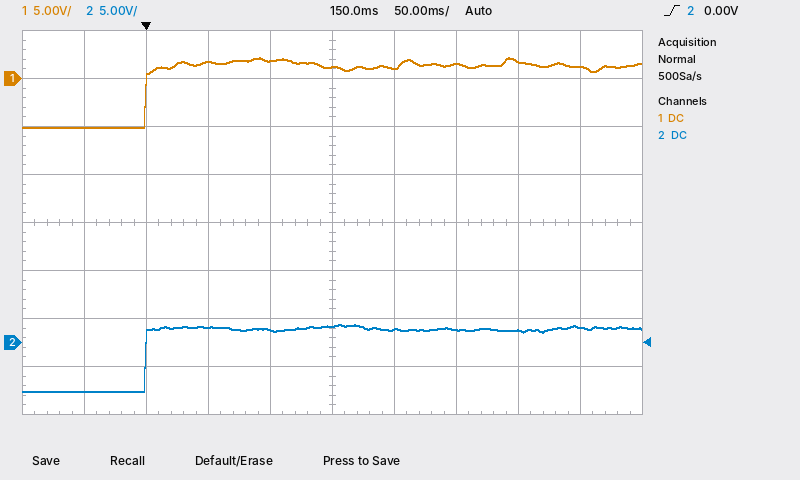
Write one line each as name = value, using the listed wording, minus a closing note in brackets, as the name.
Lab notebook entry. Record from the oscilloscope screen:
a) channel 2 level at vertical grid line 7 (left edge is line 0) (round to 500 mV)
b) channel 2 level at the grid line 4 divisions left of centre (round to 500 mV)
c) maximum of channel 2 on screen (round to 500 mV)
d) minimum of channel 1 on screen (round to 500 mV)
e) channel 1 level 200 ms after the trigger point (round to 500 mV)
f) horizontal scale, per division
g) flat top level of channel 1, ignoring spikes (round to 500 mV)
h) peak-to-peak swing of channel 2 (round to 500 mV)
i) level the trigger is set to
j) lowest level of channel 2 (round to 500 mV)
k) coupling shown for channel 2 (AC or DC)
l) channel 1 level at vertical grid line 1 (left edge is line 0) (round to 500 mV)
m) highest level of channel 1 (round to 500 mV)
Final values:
channel 2 level at vertical grid line 7 (left edge is line 0) = 1.5 V
channel 2 level at the grid line 4 divisions left of centre = -5.0 V
maximum of channel 2 on screen = 2.0 V
minimum of channel 1 on screen = -5.0 V
channel 1 level 200 ms after the trigger point = 1.0 V
horizontal scale, per division = 50 ms
flat top level of channel 1, ignoring spikes = 1.5 V
peak-to-peak swing of channel 2 = 7.0 V
level the trigger is set to = 0.00 V
lowest level of channel 2 = -5.0 V
coupling shown for channel 2 = DC
channel 1 level at vertical grid line 1 (left edge is line 0) = -5.0 V
highest level of channel 1 = 2.0 V
